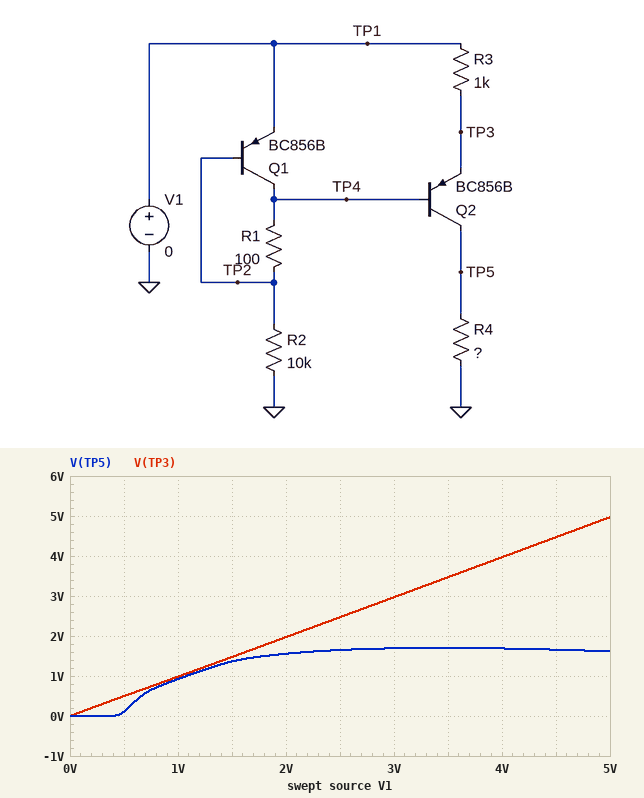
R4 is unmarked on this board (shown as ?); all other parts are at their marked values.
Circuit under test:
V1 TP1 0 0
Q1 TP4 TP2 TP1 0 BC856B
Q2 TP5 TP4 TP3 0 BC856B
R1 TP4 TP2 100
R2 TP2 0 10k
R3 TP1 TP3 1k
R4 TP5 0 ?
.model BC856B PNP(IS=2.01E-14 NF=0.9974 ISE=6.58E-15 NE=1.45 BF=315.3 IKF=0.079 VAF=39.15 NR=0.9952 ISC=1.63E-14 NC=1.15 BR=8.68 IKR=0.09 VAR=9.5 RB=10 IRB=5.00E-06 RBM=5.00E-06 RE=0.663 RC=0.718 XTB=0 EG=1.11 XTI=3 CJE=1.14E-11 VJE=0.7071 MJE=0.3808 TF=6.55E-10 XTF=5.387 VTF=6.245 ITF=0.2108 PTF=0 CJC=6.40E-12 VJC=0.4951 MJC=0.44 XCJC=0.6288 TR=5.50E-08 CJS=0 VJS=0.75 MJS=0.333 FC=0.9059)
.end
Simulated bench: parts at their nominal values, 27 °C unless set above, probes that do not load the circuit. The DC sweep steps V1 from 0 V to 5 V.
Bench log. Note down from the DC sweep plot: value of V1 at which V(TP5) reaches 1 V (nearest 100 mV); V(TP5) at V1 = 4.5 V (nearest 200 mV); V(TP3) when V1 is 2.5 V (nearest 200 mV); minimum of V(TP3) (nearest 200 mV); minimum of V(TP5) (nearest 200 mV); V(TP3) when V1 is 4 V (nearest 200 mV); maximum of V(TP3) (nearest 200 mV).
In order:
1.1 V
1.6 V
2.4 V
0 V
0 V
4.0 V
5.0 V
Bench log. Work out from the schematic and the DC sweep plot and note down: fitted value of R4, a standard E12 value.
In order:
56 kΩ
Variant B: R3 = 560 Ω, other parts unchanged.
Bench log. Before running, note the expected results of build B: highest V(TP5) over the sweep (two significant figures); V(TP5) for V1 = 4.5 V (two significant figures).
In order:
2.3 V
2.2 V
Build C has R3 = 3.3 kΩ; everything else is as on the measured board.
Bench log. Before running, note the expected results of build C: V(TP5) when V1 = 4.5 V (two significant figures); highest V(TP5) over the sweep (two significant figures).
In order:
820 mV
840 mV
